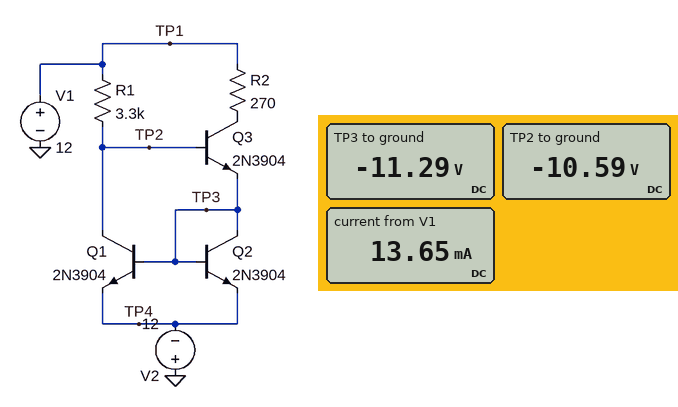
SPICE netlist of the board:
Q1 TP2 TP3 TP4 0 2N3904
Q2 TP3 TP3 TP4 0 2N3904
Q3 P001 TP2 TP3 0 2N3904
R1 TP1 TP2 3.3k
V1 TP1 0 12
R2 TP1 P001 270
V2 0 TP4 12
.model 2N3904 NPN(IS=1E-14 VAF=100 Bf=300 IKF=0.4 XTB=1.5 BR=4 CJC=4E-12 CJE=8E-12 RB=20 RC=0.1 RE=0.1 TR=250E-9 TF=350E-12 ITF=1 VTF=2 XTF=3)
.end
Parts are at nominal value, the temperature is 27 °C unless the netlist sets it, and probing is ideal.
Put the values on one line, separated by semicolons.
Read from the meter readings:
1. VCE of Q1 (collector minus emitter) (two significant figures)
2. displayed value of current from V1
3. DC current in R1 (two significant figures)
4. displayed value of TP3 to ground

1.4 V; 13.65 mA; 6.8 mA; -11.29 V
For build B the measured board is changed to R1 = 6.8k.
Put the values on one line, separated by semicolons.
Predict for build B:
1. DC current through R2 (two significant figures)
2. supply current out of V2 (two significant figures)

3.3 mA; 6.6 mA
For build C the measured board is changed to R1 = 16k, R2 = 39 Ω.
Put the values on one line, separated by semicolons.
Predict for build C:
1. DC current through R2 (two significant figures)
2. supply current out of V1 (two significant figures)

1.4 mA; 2.8 mA
